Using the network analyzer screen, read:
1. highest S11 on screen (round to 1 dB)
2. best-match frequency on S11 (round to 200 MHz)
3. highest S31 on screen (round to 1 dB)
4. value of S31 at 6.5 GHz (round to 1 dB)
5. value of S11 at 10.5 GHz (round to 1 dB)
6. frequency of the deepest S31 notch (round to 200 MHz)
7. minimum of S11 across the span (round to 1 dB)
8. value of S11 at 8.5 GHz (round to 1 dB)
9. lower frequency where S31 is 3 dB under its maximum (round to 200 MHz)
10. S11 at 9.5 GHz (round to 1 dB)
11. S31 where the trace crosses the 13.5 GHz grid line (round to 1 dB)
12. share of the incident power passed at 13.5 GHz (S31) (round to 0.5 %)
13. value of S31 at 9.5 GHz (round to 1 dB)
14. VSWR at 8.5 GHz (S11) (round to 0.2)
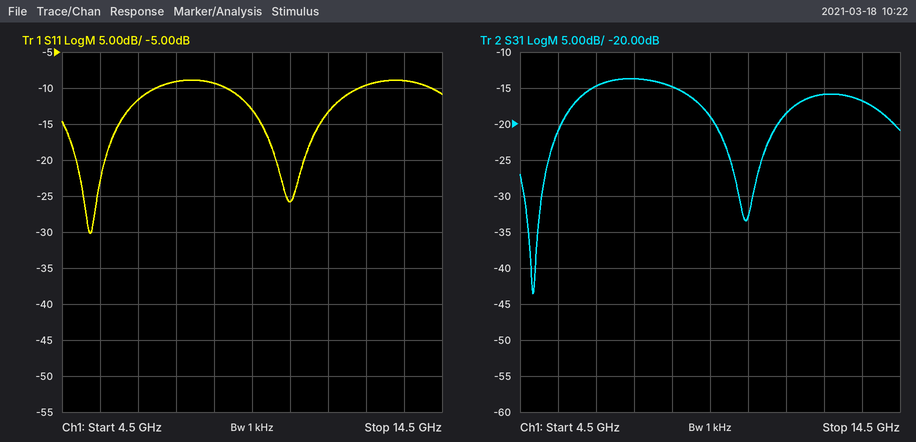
-9 dB
5.2 GHz
-14 dB
-15 dB
-26 dB
4.8 GHz
-30 dB
-9 dB
6.0 GHz
-13 dB
-17 dB
2.0 %
-19 dB
2.0
